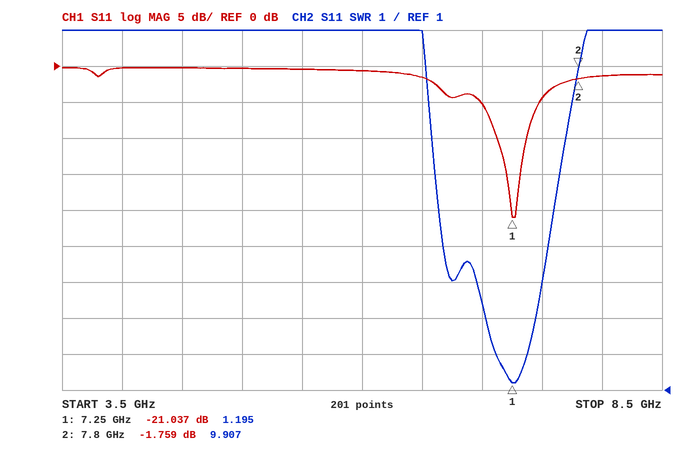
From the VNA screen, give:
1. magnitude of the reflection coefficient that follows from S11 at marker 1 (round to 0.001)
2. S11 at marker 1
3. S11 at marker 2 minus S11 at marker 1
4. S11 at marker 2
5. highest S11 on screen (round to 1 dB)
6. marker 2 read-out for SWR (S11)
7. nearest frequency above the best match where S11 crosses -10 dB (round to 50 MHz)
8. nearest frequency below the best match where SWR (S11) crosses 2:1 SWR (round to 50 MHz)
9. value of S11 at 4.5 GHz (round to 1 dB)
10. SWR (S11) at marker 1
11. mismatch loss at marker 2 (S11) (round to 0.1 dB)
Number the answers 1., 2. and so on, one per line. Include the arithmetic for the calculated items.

1. 10^(-21.037/20) ≈ 0.089
2. -21.037 dB
3. -1.759 − (-21.037) = 19.278 dB
4. -1.759 dB
5. 0 dB
6. 9.907
7. 7.35 GHz
8. 7.10 GHz
9. 0 dB
10. 1.195
11. −10 log10(1 − 10^(-1.759/10)) ≈ 4.8 dB
